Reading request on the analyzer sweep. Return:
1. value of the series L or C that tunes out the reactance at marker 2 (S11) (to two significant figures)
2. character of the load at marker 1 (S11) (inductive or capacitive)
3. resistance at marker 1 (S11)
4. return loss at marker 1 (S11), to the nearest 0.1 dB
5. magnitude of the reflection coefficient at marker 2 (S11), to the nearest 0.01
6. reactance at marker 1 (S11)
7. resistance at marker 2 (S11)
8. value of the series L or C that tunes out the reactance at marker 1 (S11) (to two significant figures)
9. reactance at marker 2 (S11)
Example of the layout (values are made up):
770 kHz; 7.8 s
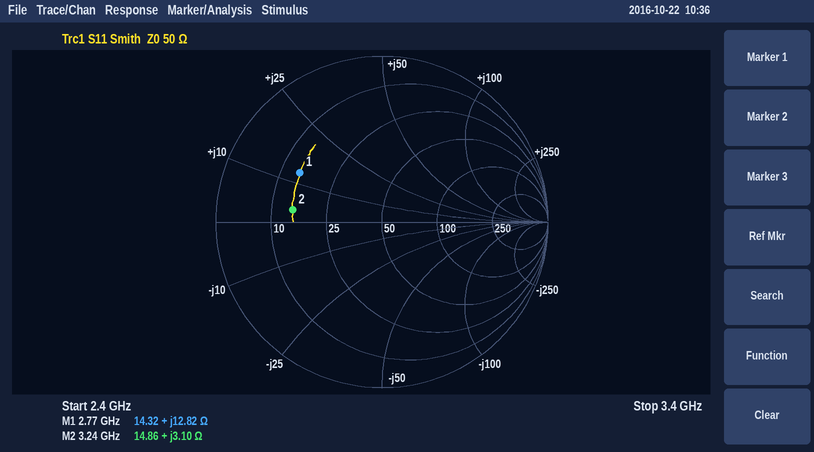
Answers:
16 pF; inductive; 14.32 Ω; 4.8 dB; 0.54; +12.82 Ω; 14.86 Ω; 4.5 pF; +3.10 Ω
